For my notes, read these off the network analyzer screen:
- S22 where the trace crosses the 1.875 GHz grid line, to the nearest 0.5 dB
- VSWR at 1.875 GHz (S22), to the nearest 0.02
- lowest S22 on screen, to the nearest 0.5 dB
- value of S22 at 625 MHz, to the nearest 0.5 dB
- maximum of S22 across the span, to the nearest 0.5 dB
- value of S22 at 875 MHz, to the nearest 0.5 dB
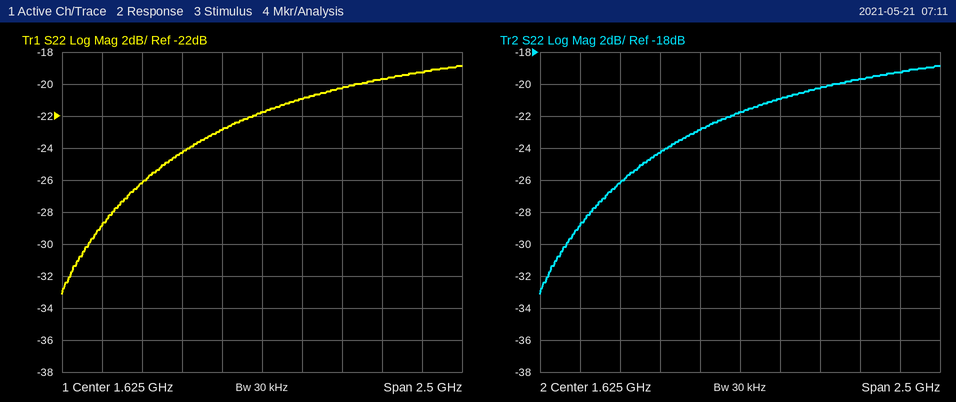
-21.0 dB
1.20
-33.0 dB
-29.0 dB
-19.0 dB
-26.0 dB
